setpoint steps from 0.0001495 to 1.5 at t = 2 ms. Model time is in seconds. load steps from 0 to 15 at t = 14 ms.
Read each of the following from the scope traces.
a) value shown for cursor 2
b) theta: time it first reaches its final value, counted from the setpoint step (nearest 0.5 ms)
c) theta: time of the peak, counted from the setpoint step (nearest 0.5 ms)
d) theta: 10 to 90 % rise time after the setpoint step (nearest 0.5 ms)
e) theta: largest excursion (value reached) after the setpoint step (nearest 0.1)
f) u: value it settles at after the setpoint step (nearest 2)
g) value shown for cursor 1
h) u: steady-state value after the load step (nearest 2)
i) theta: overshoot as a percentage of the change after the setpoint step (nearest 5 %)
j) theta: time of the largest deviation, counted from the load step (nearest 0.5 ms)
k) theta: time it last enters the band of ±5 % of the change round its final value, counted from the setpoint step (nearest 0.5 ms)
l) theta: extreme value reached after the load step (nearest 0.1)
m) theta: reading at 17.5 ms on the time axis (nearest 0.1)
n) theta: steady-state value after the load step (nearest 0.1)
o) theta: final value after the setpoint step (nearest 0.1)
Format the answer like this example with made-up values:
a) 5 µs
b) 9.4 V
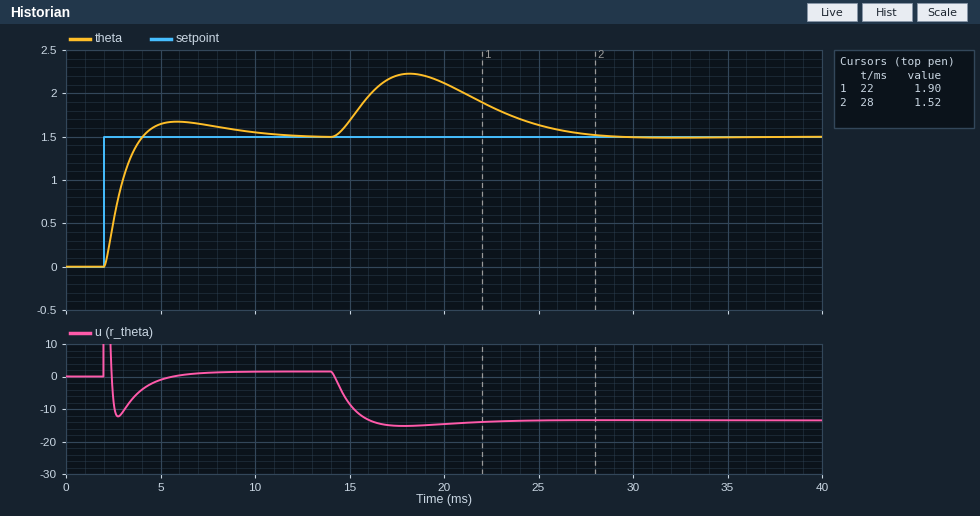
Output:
a) 1.52
b) 2.0 ms
c) 4.0 ms
d) 1.5 ms
e) 1.7
f) 2
g) 1.90
h) -14
i) 10 %
j) 4.0 ms
k) 7.0 ms
l) 2.2
m) 2.2
n) 1.5
o) 1.5
